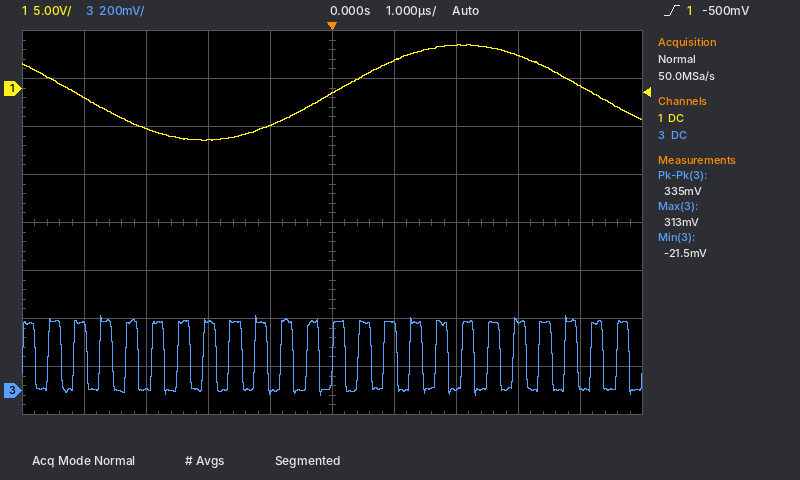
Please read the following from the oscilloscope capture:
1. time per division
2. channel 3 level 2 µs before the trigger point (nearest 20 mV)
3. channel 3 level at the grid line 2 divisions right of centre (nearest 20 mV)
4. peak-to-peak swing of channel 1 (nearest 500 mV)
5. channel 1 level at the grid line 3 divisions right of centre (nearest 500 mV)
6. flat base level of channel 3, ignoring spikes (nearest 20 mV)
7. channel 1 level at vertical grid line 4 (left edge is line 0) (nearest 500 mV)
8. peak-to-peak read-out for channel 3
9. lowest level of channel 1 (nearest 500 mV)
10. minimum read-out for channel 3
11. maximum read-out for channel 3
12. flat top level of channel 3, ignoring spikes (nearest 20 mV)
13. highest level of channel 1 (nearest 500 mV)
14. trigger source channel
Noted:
1 µs
280 mV
0 mV
10.0 V
3.5 V
0 mV
-4.0 V
335 mV
-5.5 V
-21.5 mV
313 mV
280 mV
4.5 V
channel 1
